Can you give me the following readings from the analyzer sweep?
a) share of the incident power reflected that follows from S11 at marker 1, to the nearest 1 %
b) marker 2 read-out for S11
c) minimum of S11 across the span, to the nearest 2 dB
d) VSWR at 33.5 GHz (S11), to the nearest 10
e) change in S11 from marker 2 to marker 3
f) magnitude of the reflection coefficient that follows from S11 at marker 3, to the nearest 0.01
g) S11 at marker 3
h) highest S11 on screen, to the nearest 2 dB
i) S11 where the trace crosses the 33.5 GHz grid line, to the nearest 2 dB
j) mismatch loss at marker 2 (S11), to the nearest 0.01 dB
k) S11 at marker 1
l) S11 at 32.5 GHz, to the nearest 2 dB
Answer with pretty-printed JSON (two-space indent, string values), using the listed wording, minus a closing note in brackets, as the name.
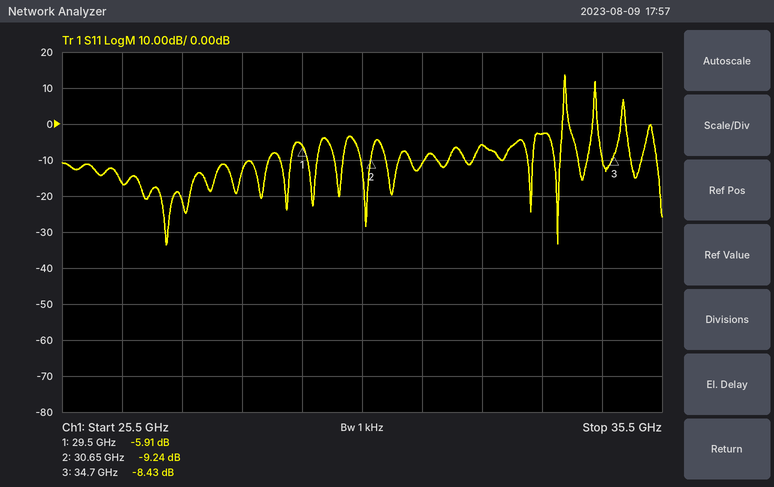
{
  "share of the incident power reflected that follows from S11 at marker 1, to the nearest 1 %": "26 %",
  "marker 2 read-out for S11": "-9.24 dB",
  "minimum of S11 across the span, to the nearest 2 dB": "-34 dB",
  "VSWR at 33.5 GHz (S11), to the nearest 10": "10",
  "change in S11 from marker 2 to marker 3": "0.81 dB",
  "magnitude of the reflection coefficient that follows from S11 at marker 3, to the nearest 0.01": "0.38",
  "S11 at marker 3": "-8.43 dB",
  "highest S11 on screen, to the nearest 2 dB": "14 dB",
  "S11 where the trace crosses the 33.5 GHz grid line, to the nearest 2 dB": "-2 dB",
  "mismatch loss at marker 2 (S11), to the nearest 0.01 dB": "0.55 dB",
  "S11 at marker 1": "-5.91 dB",
  "S11 at 32.5 GHz, to the nearest 2 dB": "-6 dB"
}
